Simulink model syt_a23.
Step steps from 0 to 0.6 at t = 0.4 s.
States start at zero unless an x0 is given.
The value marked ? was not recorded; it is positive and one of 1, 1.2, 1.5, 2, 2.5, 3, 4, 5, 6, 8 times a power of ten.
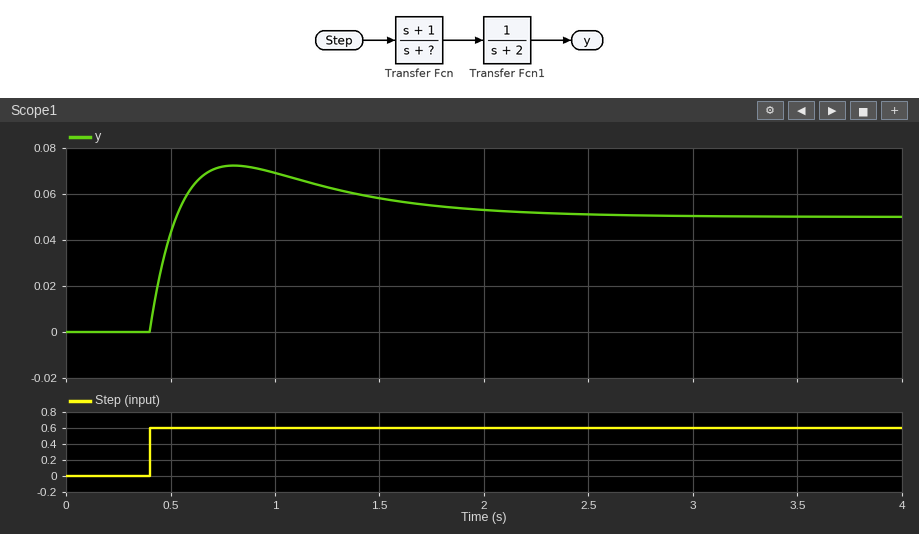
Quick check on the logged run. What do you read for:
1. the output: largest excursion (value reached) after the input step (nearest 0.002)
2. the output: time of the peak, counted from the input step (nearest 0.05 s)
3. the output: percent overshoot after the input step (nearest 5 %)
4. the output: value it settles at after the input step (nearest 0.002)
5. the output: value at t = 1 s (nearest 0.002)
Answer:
0.072
0.40 s
45 %
0.050
0.070
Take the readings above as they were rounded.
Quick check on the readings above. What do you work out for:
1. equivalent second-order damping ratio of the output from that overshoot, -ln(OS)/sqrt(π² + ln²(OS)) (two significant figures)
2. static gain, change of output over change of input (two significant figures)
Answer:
0.25
0.083
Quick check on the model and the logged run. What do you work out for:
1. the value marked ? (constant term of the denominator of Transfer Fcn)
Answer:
6
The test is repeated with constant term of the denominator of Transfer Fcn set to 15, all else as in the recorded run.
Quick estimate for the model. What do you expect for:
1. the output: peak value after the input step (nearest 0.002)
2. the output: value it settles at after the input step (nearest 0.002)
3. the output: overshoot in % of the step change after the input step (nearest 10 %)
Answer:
0.034
0.020
70 %
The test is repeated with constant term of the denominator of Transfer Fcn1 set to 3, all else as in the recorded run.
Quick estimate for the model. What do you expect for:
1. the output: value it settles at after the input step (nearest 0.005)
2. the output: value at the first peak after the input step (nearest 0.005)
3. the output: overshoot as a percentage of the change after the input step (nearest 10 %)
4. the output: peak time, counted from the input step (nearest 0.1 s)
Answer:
0.035
0.060
80 %
0.3 s
